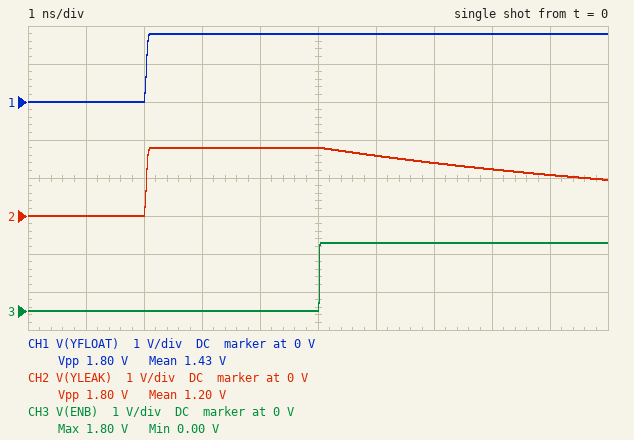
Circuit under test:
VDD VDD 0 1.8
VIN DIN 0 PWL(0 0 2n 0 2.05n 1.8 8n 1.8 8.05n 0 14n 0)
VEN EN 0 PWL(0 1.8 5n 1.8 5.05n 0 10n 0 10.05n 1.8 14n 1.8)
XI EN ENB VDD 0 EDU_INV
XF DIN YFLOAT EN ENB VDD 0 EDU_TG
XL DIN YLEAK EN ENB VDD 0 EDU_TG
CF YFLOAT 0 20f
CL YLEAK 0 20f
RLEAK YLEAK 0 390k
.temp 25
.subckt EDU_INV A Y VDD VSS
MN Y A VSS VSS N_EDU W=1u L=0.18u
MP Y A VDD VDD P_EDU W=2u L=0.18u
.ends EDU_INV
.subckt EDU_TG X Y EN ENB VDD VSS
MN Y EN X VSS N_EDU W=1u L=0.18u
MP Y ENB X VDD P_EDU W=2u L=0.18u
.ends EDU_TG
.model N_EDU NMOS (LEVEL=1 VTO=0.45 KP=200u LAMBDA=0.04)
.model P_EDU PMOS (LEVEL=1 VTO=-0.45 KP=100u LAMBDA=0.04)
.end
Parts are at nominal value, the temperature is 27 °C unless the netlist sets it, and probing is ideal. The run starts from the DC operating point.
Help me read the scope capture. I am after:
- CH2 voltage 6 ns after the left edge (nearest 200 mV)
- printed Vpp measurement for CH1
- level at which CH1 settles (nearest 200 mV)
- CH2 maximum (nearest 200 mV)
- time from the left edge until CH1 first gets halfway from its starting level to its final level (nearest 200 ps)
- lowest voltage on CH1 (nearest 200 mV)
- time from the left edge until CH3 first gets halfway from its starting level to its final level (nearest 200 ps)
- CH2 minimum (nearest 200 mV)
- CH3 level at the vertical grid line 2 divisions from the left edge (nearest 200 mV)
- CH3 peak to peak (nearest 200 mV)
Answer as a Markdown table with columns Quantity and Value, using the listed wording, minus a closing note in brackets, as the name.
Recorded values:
| Quantity | Value |
|---|---|
| CH2 voltage 6 ns after the left edge | 1.6 V |
| printed Vpp measurement for CH1 | 1.80 V |
| level at which CH1 settles | 1.8 V |
| CH2 maximum | 1.8 V |
| time from the left edge until CH1 first gets halfway from its starting level to its final level | 2.0 ns |
| lowest voltage on CH1 | 0 V |
| time from the left edge until CH3 first gets halfway from its starting level to its final level | 5.0 ns |
| CH2 minimum | 0 V |
| CH3 level at the vertical grid line 2 divisions from the left edge | 0 V |
| CH3 peak to peak | 1.8 V |
